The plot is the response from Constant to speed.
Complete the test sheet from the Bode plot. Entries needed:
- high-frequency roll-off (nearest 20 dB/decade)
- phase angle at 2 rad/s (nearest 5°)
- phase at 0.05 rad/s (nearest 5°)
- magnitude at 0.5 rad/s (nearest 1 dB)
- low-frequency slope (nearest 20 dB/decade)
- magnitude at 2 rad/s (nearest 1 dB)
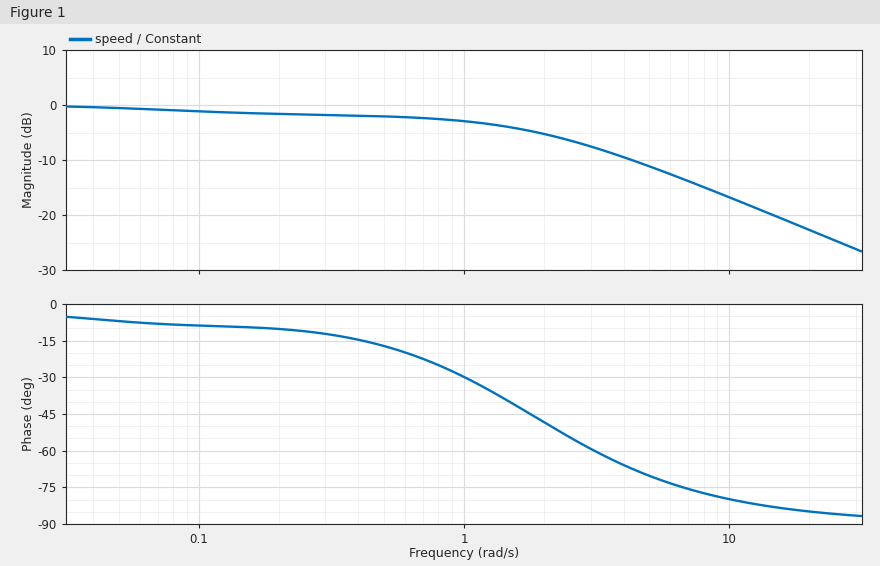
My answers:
-20 dB/decade
-50°
-5°
-2 dB
0 dB/decade
-5 dB
